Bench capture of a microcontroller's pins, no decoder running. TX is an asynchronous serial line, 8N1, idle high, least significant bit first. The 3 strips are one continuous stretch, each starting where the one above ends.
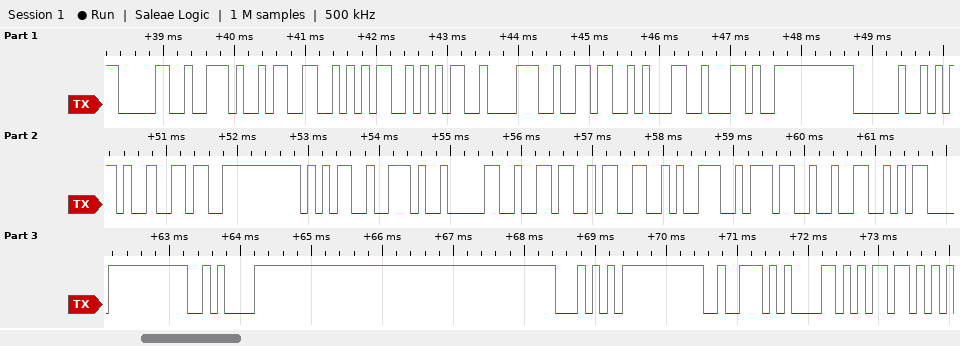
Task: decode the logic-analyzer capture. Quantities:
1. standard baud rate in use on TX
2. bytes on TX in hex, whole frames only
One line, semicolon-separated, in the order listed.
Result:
9600 baud; 30 2E 33 35 35 38 36 31 2C 20 2D 36 35 2E 30 36 33 39 37 32 0D 0A 54 72 61 6D
